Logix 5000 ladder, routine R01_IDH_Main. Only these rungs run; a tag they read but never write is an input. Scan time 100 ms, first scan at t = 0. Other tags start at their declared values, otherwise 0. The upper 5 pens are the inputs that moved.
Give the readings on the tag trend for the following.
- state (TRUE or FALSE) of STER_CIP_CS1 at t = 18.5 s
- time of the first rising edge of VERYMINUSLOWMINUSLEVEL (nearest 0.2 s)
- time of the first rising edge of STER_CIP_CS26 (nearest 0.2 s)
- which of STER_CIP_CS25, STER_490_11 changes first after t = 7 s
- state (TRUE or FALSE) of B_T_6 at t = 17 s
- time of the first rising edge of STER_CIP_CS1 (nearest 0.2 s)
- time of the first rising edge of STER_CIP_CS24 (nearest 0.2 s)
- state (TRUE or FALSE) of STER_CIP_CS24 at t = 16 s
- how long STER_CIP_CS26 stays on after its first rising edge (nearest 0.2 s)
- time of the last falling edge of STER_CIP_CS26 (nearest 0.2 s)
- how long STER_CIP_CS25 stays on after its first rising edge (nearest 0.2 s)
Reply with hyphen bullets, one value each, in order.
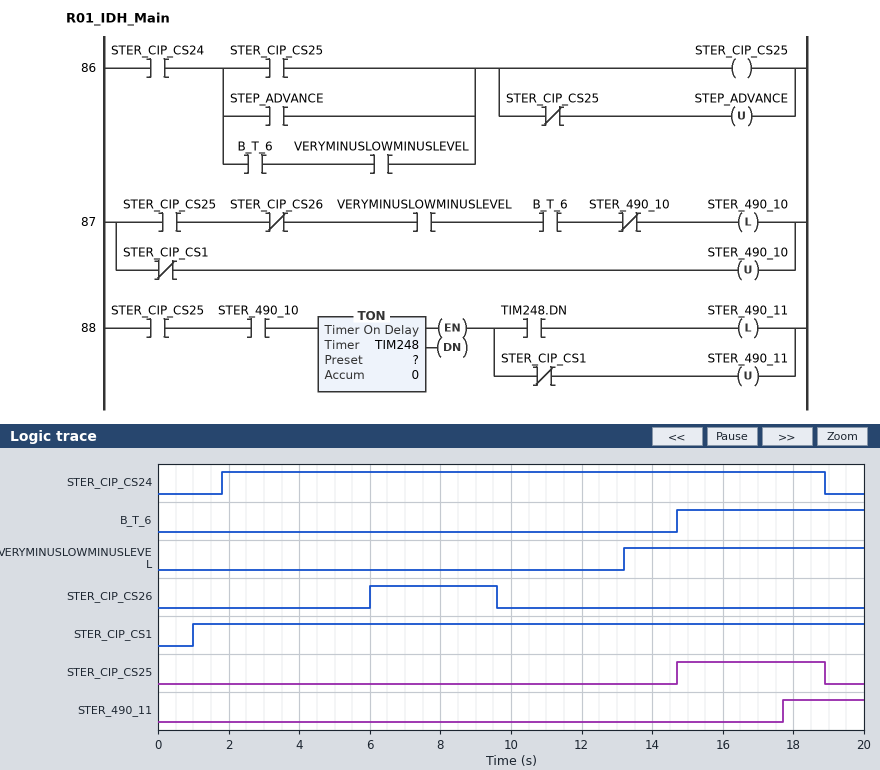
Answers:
- TRUE
- 13.2 s
- 6.0 s
- STER_CIP_CS25
- TRUE
- 1.0 s
- 1.8 s
- TRUE
- 3.6 s
- 9.6 s
- 4.2 s
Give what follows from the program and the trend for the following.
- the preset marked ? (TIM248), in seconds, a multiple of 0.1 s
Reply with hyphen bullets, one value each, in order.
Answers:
- 3.0 s
